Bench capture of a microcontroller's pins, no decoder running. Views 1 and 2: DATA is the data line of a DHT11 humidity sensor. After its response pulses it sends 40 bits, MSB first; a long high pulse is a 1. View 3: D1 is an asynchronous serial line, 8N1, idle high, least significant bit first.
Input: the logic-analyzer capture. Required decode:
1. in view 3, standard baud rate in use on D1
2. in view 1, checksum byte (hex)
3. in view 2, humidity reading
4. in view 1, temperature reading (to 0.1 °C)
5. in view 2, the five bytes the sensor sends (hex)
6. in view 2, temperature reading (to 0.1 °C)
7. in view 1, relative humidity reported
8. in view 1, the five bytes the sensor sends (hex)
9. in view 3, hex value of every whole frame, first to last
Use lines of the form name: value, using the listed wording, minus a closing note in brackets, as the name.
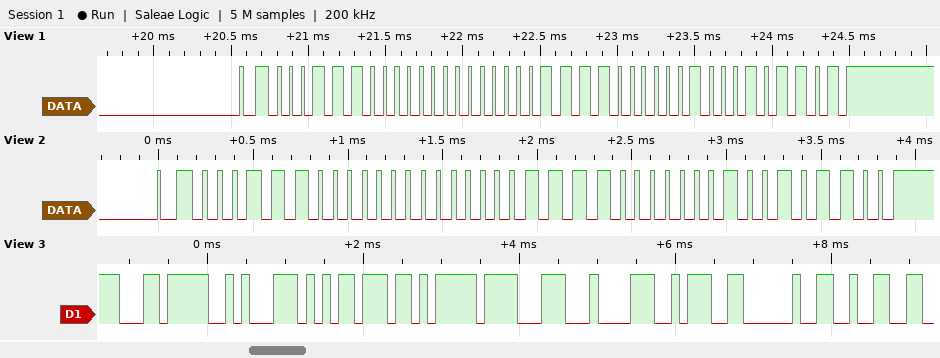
in view 3, standard baud rate in use on D1: 9600 baud
in view 1, checksum byte: 0x2D
in view 2, humidity reading: 28 %
in view 1, temperature reading: 15.2 °C
in view 2, the five bytes the sensor sends: 1C 00 0F 01 2C
in view 2, temperature reading: 15.1 °C
in view 1, relative humidity reported: 28 %
in view 1, the five bytes the sensor sends: 1C 00 0F 02 2D
in view 3, hex value of every whole frame, first to last: EC 8A B5 EB 8F 84 3A 20 32
